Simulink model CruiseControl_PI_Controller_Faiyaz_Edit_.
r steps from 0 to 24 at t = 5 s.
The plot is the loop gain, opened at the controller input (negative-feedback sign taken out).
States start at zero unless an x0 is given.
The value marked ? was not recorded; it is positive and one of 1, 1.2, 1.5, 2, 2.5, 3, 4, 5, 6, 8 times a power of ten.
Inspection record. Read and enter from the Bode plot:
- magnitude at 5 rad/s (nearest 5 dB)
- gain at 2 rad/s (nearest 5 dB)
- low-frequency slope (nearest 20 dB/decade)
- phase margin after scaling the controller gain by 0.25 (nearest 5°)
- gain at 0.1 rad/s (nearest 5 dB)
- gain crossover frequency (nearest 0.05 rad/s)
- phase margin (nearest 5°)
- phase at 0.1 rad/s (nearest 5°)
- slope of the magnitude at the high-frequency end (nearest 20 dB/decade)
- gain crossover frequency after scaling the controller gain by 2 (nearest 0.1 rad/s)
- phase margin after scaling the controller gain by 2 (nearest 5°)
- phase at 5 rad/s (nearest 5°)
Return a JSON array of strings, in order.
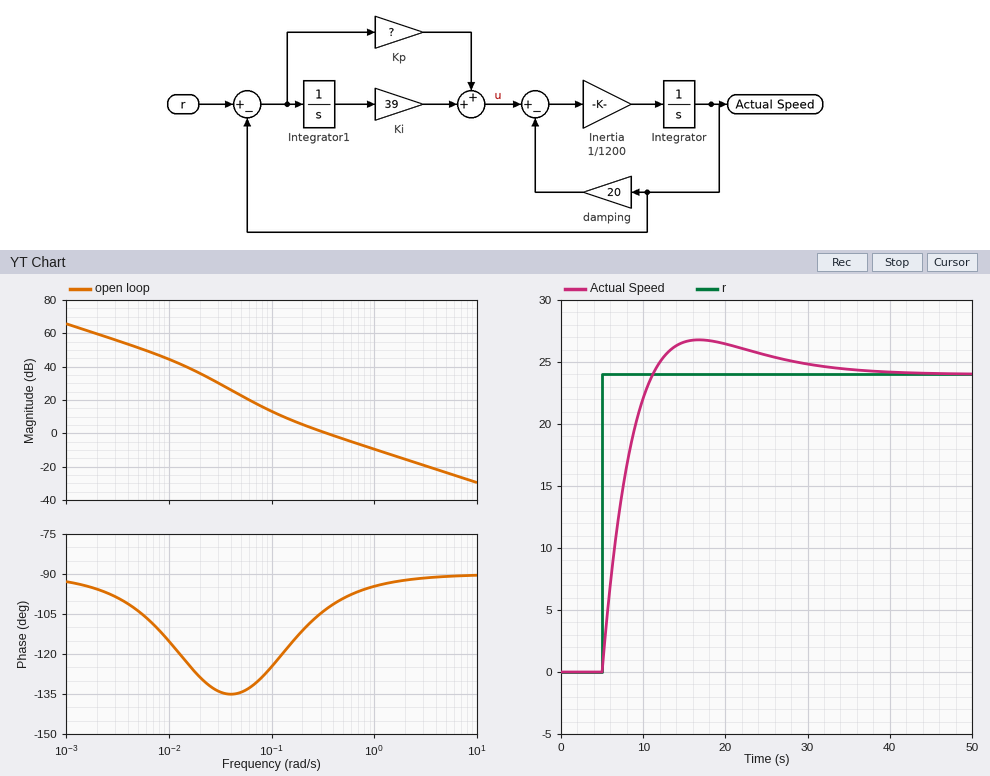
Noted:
["-25 dB", "-15 dB", "-20 dB/decade", "55°", "15 dB", "0.35 rad/s", "75°", "-125°", "-20 dB/decade", "0.7 rad/s", "85°", "-90°"]
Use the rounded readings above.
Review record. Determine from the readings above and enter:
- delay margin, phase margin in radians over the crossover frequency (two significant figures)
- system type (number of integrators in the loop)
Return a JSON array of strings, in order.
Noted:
["3.7 s", "1"]
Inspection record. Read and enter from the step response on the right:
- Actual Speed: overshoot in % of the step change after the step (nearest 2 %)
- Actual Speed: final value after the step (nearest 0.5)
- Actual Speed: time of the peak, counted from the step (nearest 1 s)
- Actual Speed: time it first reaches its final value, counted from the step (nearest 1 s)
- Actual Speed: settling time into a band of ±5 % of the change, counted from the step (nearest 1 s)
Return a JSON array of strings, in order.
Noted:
["12 %", "24.0", "12 s", "6 s", "22 s"]
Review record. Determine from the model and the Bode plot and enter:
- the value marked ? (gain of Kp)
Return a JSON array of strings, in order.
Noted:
["400"]
